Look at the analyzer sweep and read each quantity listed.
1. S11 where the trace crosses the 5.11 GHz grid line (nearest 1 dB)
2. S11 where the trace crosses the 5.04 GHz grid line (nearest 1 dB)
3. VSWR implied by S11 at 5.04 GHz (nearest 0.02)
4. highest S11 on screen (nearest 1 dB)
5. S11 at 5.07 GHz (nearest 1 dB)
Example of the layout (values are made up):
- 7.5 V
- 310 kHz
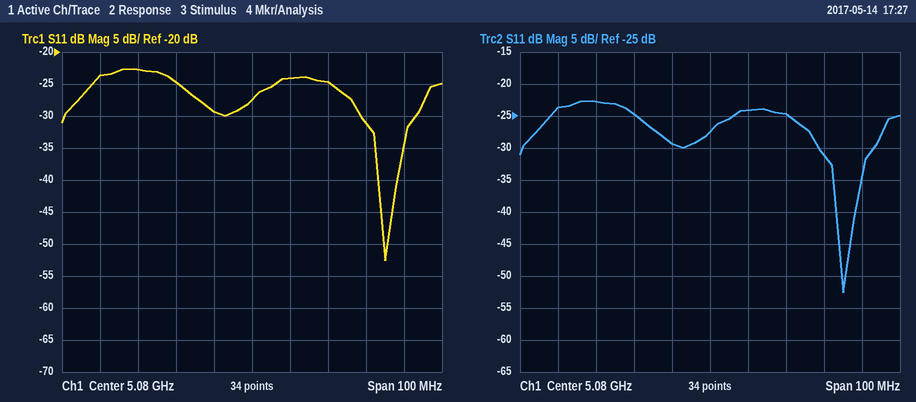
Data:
- -31 dB
- -24 dB
- 1.14
- -23 dB
- -29 dB
